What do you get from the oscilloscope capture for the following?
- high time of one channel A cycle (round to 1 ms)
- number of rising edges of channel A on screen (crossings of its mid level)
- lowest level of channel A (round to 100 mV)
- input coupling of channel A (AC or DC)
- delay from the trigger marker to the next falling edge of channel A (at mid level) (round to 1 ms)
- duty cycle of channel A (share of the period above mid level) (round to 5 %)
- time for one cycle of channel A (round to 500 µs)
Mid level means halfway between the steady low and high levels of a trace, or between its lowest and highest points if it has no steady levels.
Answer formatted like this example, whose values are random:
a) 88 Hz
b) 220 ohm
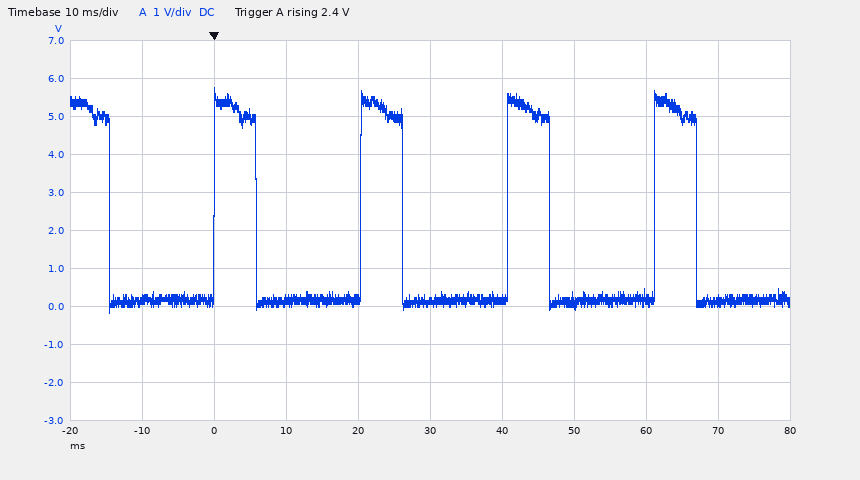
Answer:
a) 6 ms
b) 4
c) -200 mV
d) DC
e) 6 ms
f) 30 %
g) 20.5 ms
